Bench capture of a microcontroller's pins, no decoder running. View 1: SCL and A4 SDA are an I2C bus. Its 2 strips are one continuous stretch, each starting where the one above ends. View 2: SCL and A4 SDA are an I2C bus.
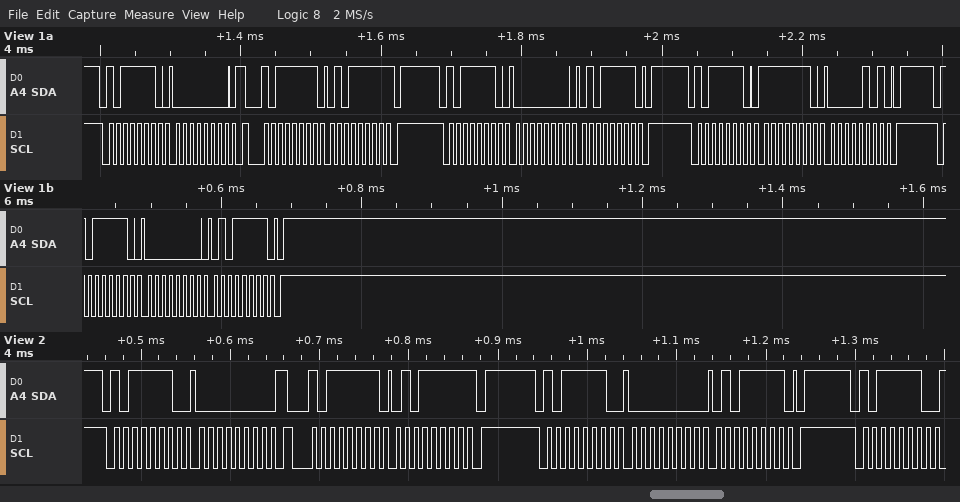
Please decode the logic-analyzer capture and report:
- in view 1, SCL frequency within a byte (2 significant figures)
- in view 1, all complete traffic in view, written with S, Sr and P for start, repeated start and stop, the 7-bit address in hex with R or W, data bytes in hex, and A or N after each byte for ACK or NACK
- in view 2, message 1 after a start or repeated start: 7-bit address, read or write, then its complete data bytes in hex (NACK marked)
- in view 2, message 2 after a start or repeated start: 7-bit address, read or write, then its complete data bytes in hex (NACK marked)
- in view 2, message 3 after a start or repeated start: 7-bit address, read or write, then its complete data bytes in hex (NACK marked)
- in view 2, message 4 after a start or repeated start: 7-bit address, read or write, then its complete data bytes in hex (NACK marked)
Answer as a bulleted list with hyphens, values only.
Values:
- 100 kHz
- S 5FW A 00 A Sr 5FR A 5F N P S 5FW A 00 A 5F A P S 5FW A FE A 05 A P S 5FW A 00 A 5F A P
- 0x5F write: 00
- 0x5F read: 5F NACK
- 0x5F write: 00 5F
- 0x5F write
